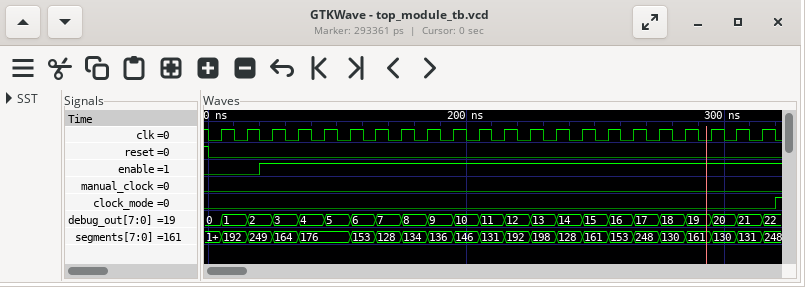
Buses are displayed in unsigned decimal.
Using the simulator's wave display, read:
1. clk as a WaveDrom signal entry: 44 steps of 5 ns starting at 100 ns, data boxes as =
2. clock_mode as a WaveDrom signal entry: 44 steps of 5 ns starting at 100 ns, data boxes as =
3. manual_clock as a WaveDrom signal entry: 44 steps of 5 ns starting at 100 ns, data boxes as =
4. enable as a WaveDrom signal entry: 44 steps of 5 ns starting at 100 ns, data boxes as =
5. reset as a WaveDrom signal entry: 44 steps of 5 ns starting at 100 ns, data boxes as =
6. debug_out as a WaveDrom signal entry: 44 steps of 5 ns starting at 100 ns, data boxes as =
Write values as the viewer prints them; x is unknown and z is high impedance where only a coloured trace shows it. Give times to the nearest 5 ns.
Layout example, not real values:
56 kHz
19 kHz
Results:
{name: 'clk', wave: '01010101010101010101010101010101010101010101'}
{name: 'clock_mode', wave: '0...........................................'}
{name: 'manual_clock', wave: '0...........................................'}
{name: 'enable', wave: '0...1.......................................'}
{name: 'reset', wave: '0...........................................'}
{name: 'debug_out', wave: '==.=.=.=.=.=.=.=.=.=.=.=.=.=.=.=.=.=.=.=.=.=', data: '0 1 2 3 4 5 6 7 8 9 10 11 12 13 14 15 16 17 18 19 20 21 22'}
